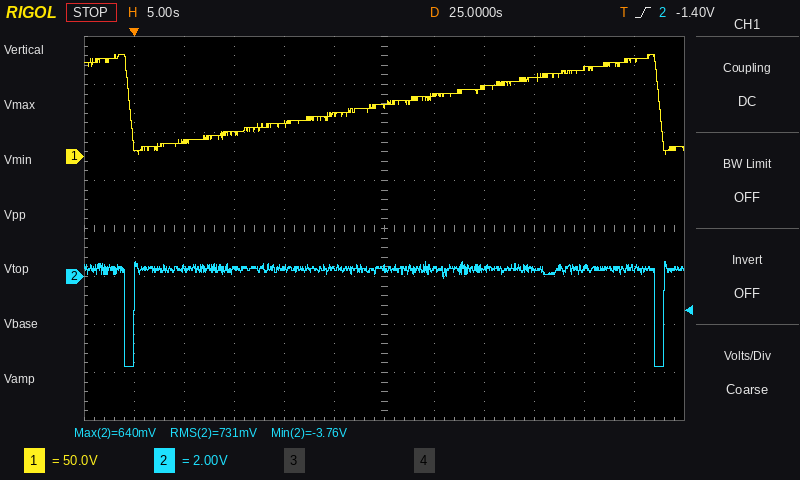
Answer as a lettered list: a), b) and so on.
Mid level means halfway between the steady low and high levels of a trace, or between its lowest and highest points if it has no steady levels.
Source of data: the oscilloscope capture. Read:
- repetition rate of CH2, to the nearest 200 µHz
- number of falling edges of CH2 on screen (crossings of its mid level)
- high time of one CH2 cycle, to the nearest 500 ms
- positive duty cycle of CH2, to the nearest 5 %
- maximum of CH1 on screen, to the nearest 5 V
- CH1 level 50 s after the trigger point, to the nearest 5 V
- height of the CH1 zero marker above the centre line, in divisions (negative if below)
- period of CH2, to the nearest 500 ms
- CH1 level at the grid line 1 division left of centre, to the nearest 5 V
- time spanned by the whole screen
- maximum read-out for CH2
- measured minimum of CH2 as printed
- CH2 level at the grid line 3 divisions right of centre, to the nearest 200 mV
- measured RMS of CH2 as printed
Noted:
a) 18.8 mHz
b) 2
c) 52.0 s
d) 100 %
e) 105 V
f) 100 V
g) +1.5 div
h) 53.0 s
i) 45 V
j) 60 s
k) 640 mV
l) -3.76 V
m) 200 mV
n) 731 mV
